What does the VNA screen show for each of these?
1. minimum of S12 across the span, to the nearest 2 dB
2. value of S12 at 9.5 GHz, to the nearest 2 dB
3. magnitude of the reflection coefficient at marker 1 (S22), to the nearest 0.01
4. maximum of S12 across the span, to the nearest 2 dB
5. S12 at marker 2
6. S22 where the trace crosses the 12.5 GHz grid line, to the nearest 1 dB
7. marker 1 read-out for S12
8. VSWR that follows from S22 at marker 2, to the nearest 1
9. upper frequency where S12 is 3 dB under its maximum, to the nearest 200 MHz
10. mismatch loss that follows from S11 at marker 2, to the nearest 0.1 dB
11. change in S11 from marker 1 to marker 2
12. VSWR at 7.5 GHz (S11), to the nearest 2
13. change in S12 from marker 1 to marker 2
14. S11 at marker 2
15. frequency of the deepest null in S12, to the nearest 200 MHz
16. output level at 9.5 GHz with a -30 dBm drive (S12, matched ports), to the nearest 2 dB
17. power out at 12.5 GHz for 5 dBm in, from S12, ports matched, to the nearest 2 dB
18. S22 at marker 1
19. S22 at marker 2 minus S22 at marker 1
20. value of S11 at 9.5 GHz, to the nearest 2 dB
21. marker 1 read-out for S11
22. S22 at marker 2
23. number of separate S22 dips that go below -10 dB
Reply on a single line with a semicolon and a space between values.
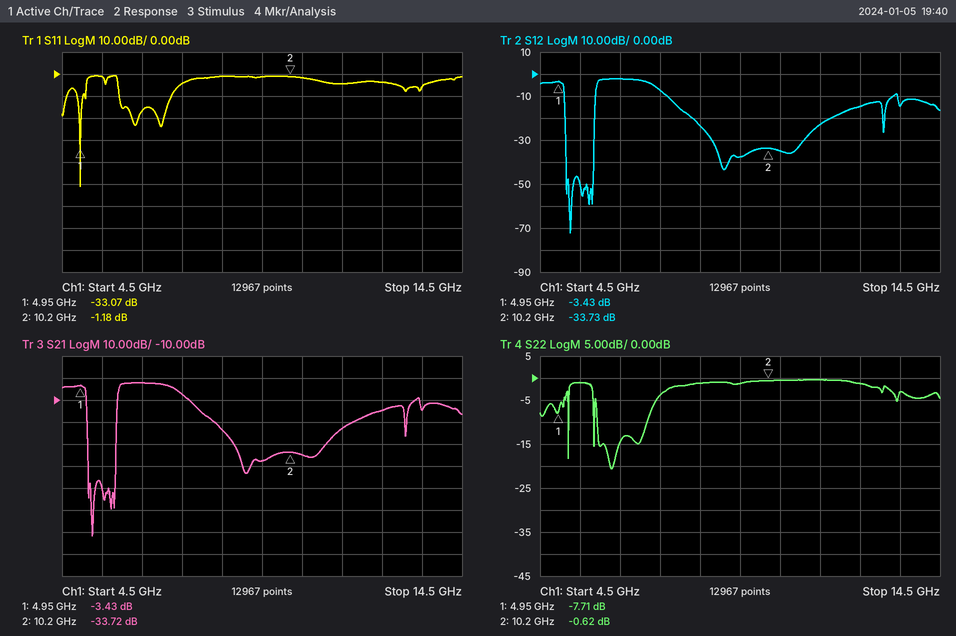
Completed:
-72 dB; -38 dB; 0.41; -2 dB; -33.73 dB; -1 dB; -3.43 dB; 28; 7.4 GHz; 6.2 dB; 31.89 dB; 4; -30.30 dB; -1.18 dB; 5.2 GHz; -68 dBm; -10 dBm; -7.71 dB; 7.09 dB; -2 dB; -33.07 dB; -0.62 dB; 3
